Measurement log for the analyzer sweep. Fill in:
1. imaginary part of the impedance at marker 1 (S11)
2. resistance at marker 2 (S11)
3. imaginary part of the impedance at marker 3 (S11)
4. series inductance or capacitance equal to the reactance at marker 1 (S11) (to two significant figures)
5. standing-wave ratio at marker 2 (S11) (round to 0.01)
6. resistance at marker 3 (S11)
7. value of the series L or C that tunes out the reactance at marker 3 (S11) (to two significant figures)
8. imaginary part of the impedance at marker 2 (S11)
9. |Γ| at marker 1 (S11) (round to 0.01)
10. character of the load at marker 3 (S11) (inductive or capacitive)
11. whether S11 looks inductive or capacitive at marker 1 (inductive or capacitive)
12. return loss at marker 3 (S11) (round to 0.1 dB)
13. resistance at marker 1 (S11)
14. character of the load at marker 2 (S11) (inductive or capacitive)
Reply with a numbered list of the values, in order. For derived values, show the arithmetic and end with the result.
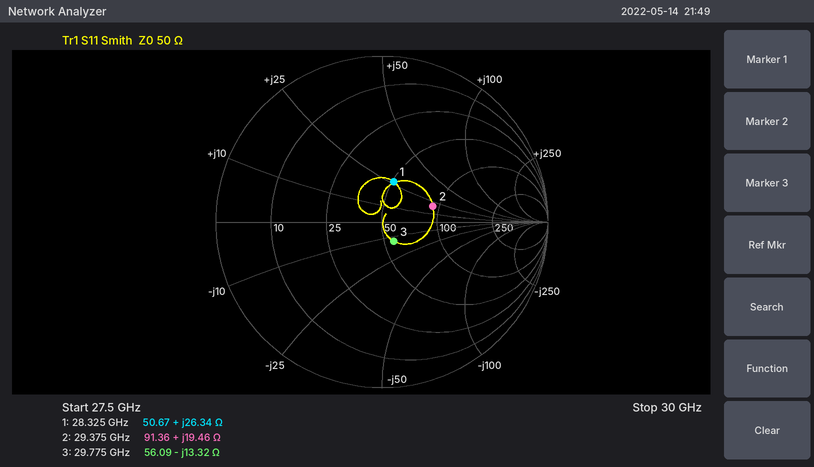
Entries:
1. +26.34 Ω
2. 91.36 Ω
3. -13.32 Ω
4. L = 26.34 Ω/(2π × 28.325 GHz) ≈ 148 pH, so 150 pH to two significant figures
5. 1.94
6. 56.09 Ω
7. L = 13.32 Ω/(2π × 29.775 GHz) ≈ 71 pH
8. +19.46 Ω
9. 0.25
10. capacitive
11. inductive
12. 17.3 dB
13. 50.67 Ω
14. inductive
